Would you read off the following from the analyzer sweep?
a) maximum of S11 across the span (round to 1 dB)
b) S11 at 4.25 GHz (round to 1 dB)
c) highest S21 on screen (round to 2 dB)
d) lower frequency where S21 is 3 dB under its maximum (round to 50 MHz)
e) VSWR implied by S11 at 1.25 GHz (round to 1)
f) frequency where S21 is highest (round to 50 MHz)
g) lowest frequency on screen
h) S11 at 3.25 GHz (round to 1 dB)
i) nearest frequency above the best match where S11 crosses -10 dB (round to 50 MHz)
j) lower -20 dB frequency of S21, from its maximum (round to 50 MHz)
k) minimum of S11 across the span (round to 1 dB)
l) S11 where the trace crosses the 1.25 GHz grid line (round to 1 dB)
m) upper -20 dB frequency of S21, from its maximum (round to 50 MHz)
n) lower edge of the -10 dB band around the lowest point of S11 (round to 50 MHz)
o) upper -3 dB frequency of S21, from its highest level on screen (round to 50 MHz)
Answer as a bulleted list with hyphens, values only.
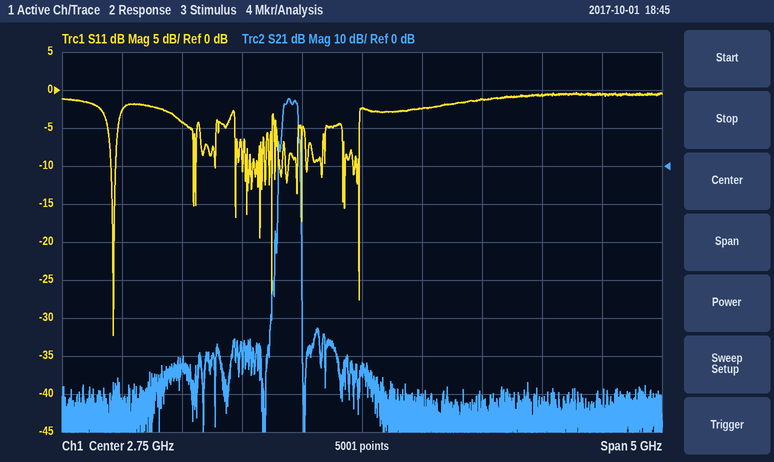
- 0 dB
- -1 dB
- 18 dB
- 2.10 GHz
- 4
- 2.15 GHz
- 250 MHz
- -2 dB
- 700 MHz
- 2.05 GHz
- -32 dB
- -4 dB
- 2.25 GHz
- 650 MHz
- 2.20 GHz
